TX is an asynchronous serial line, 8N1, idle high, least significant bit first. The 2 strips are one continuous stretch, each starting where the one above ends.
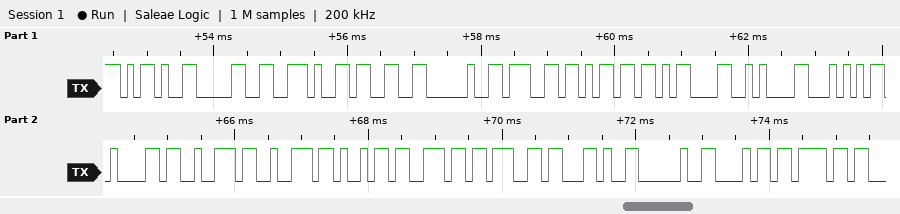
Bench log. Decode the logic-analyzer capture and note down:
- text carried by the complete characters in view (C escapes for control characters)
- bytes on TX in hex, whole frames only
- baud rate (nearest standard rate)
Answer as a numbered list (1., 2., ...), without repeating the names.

1. "-0.3 gm\r\nTarring, ho"
2. 0x2D 0x30 0x2E 0x33 0x20 0x67 0x6D 0x0D 0x0A 0x54 0x61 0x72 0x72 0x69 0x6E 0x67 0x2C 0x20 0x68 0x6F
3. 9600 baud
